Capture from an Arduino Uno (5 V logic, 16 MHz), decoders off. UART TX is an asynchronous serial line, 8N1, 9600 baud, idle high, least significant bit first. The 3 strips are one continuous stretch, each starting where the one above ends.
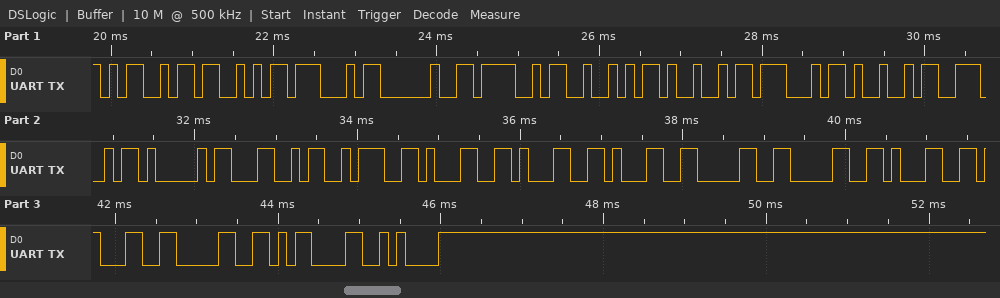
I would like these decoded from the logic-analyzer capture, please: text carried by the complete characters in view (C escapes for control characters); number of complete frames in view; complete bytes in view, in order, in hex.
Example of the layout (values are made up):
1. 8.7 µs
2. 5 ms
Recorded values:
1. "MSG ORIGINAL:11100110\r\n"
2. 23
3. 4D 53 47 20 4F 52 49 47 49 4E 41 4C 3A 31 31 31 30 30 31 31 30 0D 0A
